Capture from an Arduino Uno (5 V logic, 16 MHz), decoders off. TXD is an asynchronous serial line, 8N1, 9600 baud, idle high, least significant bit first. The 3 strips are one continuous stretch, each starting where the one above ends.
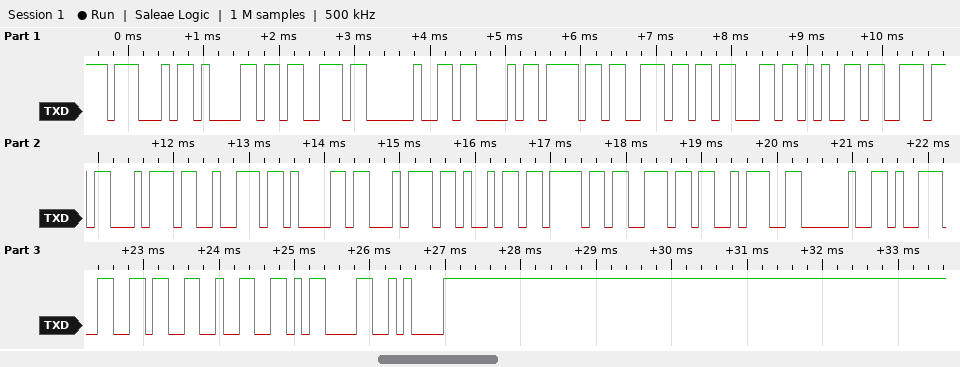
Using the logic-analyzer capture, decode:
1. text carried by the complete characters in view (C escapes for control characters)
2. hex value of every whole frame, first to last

"Gas Concentration: 962\r\n"
47 61 73 20 43 6F 6E 63 65 6E 74 72 61 74 69 6F 6E 3A 20 39 36 32 0D 0A
